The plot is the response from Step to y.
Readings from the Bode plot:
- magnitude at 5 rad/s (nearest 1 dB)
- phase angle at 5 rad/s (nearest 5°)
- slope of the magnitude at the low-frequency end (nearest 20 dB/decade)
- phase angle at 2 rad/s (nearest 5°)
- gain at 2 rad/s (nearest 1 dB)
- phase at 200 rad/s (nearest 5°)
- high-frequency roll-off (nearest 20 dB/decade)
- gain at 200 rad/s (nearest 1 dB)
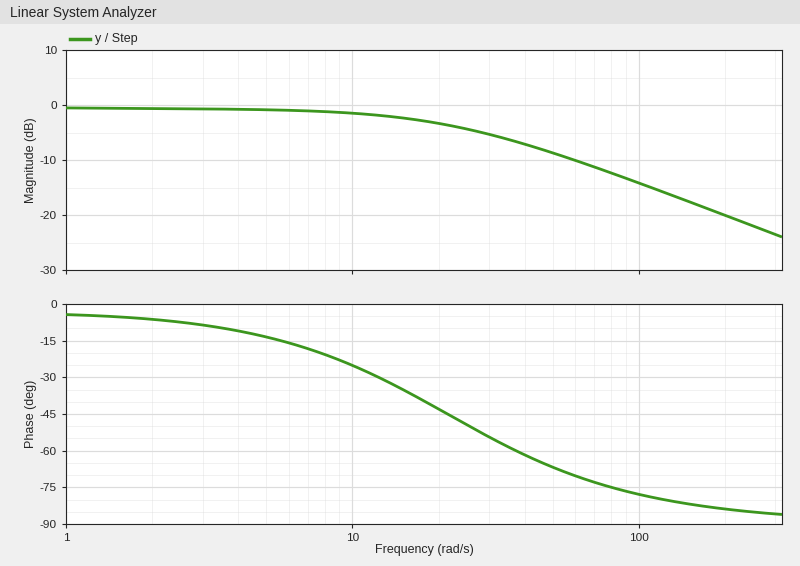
-1 dB
-15°
0 dB/decade
-5°
-1 dB
-85°
-20 dB/decade
-20 dB
